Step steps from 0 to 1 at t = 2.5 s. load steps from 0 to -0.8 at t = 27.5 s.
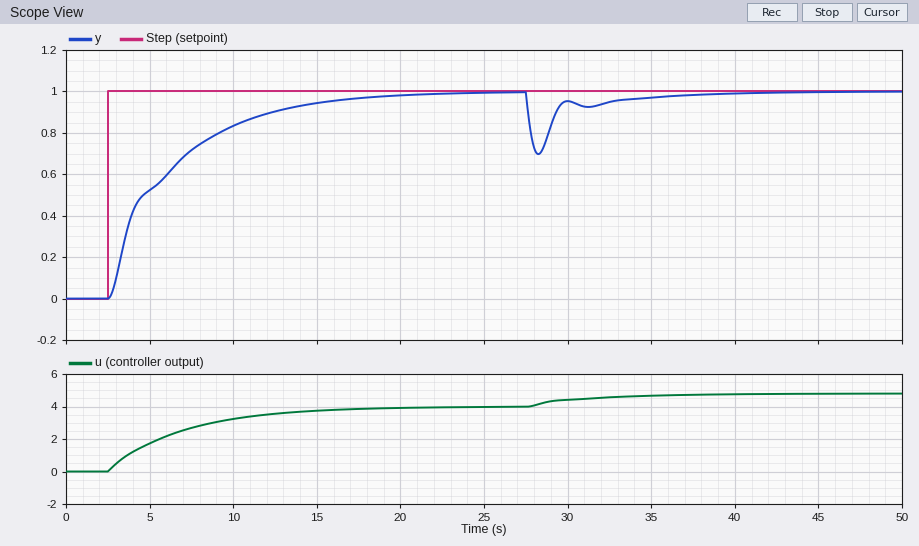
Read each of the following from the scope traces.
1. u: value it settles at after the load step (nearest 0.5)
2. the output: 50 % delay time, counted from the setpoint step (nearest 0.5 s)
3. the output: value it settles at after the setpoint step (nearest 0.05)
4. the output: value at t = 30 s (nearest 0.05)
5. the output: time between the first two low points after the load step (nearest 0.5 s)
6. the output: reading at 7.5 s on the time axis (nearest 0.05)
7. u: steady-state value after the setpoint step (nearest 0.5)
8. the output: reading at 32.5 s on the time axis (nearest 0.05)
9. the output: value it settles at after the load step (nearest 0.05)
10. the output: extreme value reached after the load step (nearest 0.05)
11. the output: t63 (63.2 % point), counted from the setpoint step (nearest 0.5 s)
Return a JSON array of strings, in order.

["5.0", "2.0 s", "1.00", "0.95", "3.0 s", "0.70", "4.0", "0.95", "1.00", "0.70", "4.0 s"]
